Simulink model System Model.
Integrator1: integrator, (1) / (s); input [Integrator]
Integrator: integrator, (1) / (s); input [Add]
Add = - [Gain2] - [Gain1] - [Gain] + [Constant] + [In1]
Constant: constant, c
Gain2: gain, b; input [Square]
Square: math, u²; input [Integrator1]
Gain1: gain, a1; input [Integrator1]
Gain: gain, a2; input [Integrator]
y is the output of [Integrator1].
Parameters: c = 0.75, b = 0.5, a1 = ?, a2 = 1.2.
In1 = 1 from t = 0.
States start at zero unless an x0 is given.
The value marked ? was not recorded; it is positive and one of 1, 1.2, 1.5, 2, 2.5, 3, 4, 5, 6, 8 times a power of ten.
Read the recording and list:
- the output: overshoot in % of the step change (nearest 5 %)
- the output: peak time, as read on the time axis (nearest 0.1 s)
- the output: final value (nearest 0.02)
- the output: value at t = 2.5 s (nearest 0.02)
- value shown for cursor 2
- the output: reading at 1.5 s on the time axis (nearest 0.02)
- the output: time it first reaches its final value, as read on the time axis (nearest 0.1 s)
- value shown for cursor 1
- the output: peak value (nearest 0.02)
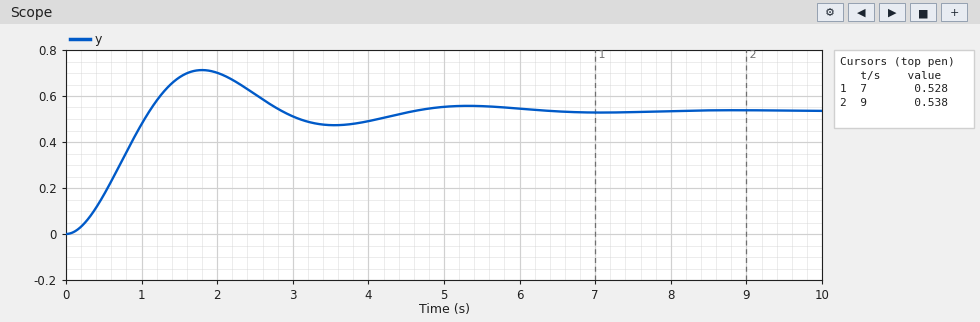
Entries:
35 %
1.8 s
0.54
0.60
0.538
0.68
1.1 s
0.528
0.72
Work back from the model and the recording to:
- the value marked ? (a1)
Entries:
3
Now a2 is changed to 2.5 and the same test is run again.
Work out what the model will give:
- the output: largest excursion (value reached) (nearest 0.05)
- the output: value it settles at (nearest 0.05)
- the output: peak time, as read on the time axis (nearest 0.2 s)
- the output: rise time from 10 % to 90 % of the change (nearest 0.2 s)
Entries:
0.55
0.55
2.4 s
1.2 s
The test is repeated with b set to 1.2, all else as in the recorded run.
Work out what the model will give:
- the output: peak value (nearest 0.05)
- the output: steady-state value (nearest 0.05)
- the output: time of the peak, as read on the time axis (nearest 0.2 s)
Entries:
0.65
0.50
1.6 s
